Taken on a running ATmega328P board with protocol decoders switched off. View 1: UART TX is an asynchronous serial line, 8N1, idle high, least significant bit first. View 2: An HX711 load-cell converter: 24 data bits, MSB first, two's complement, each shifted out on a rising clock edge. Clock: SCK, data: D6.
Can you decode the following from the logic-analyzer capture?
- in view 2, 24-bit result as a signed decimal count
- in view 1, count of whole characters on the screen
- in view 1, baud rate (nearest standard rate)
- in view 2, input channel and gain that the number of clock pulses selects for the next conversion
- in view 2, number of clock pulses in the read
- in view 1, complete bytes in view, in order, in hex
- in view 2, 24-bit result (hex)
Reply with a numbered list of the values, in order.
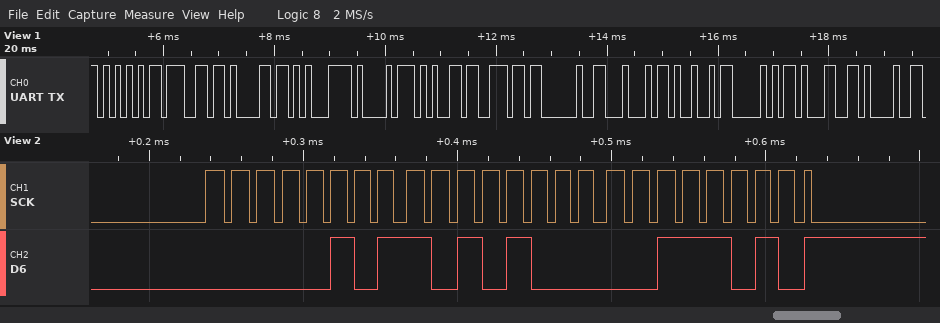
1. 370746
2. 13
3. 9600 baud
4. channel A, gain 128
5. 25
6. 55 67 61 C5 A1 65 6E 20 44 49 50 31 21
7. 0x05A83A
